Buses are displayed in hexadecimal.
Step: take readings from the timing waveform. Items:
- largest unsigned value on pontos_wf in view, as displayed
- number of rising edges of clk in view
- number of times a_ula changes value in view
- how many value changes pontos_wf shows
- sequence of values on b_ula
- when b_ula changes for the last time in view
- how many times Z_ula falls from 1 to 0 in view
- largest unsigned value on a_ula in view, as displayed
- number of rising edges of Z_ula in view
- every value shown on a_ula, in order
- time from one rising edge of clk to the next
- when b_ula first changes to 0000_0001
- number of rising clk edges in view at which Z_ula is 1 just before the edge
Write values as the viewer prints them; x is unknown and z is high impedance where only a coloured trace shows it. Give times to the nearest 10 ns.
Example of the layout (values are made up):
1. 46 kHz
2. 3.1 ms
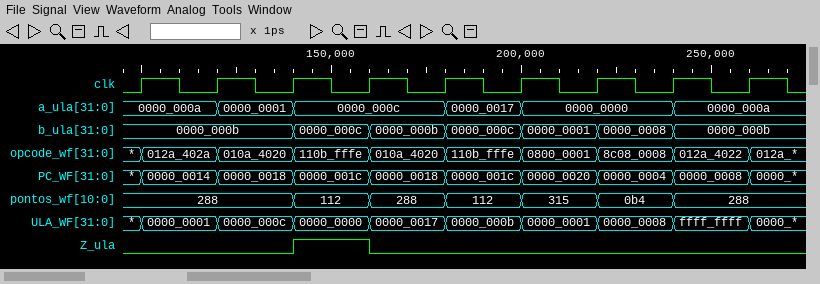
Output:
1. 315
2. 9
3. 5
4. 6
5. 0000_000b, 0000_000c, 0000_000b, 0000_000c, 0000_0001, 0000_0008, 0000_000b
6. 240 ns
7. 1
8. 0000_0017
9. 1
10. 0000_000a, 0000_0001, 0000_000c, 0000_0017, 0000_0000, 0000_000a
11. 20 ns
12. 200 ns
13. 1
